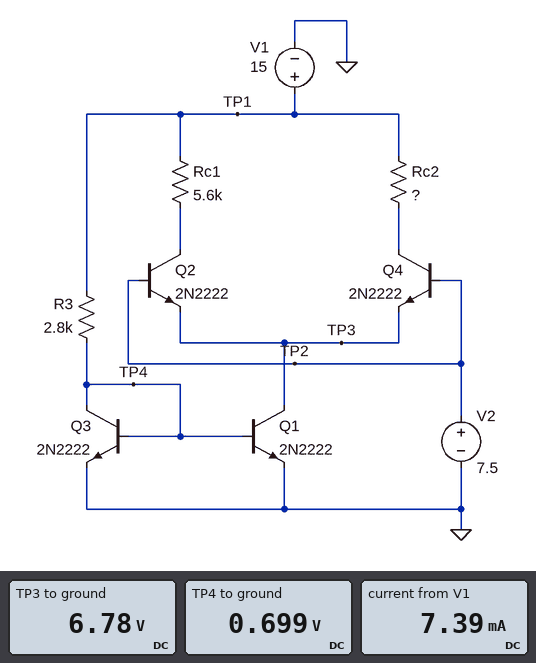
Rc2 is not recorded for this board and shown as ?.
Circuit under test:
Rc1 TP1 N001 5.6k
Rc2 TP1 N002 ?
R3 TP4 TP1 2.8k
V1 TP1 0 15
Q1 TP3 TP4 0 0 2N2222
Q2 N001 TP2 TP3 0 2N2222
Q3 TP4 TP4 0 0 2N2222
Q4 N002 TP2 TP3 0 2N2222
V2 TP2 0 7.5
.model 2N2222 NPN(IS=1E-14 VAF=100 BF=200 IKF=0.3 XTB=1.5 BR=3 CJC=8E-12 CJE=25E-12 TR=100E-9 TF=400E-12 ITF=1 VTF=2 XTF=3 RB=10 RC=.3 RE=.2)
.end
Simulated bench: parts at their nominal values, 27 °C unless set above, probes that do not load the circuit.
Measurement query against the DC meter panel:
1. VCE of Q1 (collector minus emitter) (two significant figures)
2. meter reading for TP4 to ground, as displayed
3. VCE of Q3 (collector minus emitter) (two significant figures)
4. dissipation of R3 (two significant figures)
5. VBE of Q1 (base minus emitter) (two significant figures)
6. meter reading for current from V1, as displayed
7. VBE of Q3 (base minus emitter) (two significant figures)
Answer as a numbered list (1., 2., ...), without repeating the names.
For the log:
1. 6.8 V
2. 0.699 V
3. 700 mV
4. 73 mW
5. 700 mV
6. 7.39 mA
7. 700 mV
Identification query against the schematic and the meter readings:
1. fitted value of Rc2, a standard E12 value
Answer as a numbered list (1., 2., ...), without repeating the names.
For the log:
1. 10 kΩ
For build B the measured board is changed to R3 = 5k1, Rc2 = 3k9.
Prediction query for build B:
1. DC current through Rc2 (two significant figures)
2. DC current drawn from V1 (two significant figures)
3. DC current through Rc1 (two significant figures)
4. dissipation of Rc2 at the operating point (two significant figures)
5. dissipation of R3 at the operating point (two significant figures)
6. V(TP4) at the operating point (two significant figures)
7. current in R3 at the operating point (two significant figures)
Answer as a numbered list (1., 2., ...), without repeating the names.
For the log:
1. 1.5 mA
2. 5.7 mA
3. 1.4 mA
4. 8.7 mW
5. 40 mW
6. 680 mV
7. 2.8 mA
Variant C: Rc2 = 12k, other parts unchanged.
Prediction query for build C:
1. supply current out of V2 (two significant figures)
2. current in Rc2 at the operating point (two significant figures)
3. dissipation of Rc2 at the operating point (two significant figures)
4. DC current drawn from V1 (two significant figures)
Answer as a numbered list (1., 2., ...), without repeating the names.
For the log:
1. 3.2 mA
2. 680 µA
3. 5.6 mW
4. 7.3 mA
